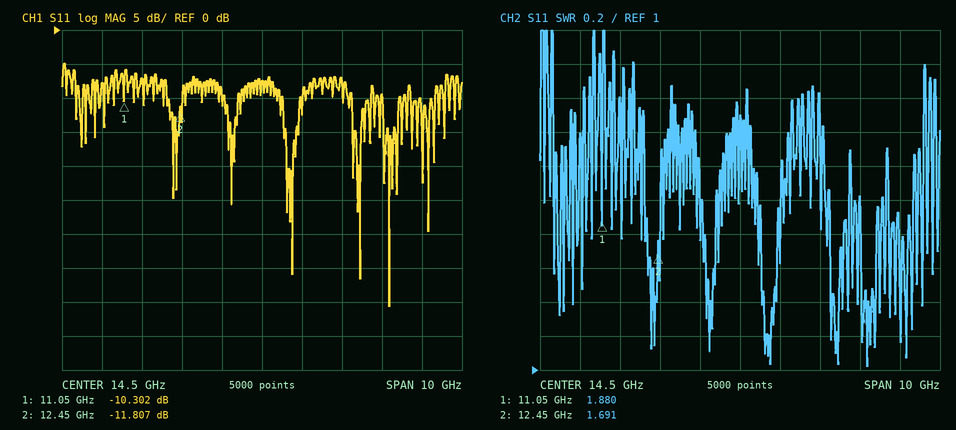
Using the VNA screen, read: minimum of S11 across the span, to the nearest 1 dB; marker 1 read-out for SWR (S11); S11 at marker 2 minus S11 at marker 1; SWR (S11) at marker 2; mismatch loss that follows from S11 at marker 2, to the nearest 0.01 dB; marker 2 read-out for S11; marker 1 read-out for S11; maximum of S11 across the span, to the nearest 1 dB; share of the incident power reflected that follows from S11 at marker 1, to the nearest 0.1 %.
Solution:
-41 dB
1.880
-1.505 dB
1.691
0.30 dB
-11.807 dB
-10.302 dB
-5 dB
9.3 %
